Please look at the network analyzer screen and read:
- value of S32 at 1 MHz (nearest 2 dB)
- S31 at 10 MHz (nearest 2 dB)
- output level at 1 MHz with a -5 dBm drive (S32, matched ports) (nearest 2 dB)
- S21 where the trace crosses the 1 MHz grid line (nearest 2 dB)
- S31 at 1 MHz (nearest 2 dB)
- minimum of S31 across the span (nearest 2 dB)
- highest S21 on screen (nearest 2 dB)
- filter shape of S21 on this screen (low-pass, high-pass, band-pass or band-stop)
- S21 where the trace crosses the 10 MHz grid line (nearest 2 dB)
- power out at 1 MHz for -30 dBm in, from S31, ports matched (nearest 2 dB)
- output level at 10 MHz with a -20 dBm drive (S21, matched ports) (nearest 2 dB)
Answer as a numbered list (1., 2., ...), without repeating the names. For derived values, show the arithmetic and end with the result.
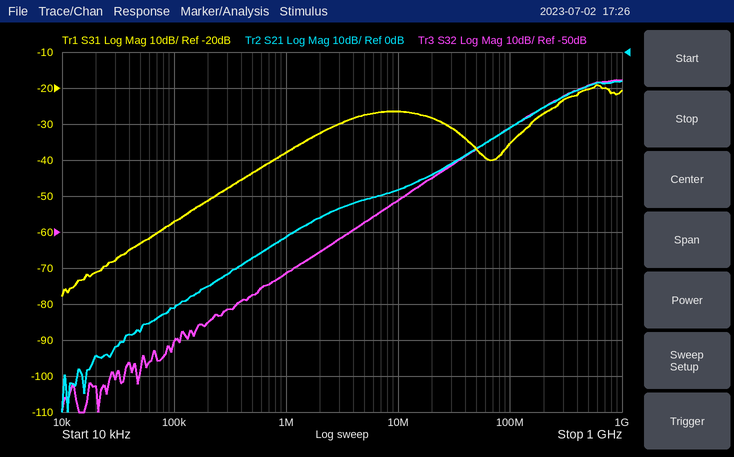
1. -62 dB
2. -26 dB
3. -5 dBm + (-62 dB) = -66 dBm
4. -52 dB
5. -38 dB
6. -78 dB
7. -8 dB
8. high-pass
9. -38 dB
10. -30 dBm + (-38 dB) = -68 dBm
11. -20 dBm + (-38 dB) = -58 dBm
